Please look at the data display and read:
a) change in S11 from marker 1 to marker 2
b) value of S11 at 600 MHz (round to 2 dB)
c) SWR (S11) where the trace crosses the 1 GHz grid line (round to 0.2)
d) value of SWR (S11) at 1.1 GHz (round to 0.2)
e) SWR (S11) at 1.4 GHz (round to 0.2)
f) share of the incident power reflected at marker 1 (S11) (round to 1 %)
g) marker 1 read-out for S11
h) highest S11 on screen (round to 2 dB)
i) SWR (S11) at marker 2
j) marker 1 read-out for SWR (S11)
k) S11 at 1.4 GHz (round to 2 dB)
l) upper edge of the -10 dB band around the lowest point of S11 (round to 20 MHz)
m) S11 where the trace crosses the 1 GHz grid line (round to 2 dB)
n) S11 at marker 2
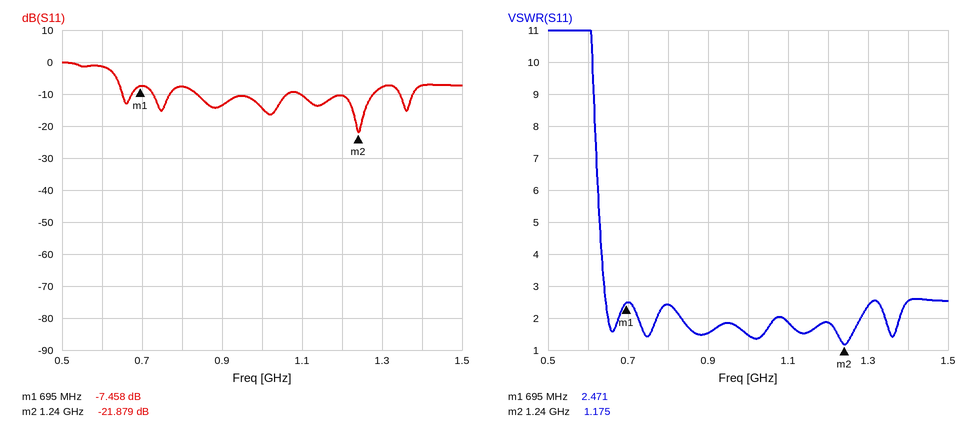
-14.421 dB
-2 dB
1.4
1.8
2.6
18 %
-7.458 dB
0 dB
1.175
2.471
-8 dB
1.28 GHz
-14 dB
-21.879 dB
